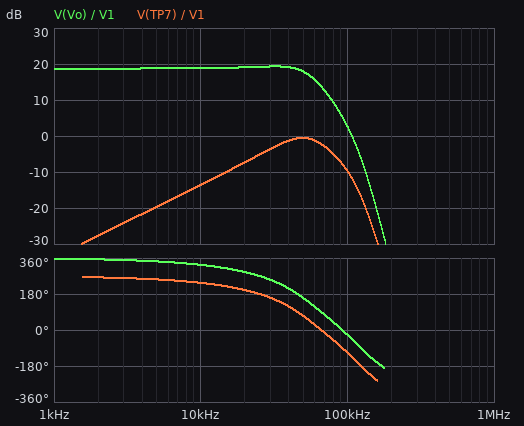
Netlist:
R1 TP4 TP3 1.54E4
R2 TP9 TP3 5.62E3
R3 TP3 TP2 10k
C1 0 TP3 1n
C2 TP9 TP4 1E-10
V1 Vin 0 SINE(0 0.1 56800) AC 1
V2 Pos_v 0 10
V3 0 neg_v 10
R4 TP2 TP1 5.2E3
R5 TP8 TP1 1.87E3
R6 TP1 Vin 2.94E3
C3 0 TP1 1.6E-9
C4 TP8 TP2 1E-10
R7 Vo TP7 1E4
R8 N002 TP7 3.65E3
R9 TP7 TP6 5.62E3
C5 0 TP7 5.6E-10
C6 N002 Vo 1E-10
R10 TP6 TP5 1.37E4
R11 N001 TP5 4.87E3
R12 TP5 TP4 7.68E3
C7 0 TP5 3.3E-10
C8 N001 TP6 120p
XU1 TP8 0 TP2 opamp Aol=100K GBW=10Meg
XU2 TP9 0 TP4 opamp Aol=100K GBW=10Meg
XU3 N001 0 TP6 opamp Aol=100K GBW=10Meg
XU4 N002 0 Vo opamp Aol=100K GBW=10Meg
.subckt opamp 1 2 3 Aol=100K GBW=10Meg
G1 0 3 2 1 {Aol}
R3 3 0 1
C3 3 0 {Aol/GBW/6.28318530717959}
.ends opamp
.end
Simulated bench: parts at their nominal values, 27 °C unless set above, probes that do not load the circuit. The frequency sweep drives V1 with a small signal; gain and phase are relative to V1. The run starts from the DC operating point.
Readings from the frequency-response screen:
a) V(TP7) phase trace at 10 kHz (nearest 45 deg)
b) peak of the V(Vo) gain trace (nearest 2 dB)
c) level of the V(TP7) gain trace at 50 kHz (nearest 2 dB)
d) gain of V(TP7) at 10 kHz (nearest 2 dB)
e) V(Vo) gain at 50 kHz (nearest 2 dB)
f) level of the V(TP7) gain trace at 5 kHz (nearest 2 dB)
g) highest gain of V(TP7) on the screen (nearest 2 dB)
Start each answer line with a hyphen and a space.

- 225 deg
- 20 dB
- 0 dB
- -14 dB
- 18 dB
- -20 dB
- 0 dB
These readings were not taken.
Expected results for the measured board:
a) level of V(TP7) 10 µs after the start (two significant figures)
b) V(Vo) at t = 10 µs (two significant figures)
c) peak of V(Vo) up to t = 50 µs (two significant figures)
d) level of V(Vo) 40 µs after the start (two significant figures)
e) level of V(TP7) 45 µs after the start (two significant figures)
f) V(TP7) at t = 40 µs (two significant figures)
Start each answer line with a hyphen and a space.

- -36 mV
- 210 mV
- 670 mV
- -490 mV
- -78 mV
- 60 mV
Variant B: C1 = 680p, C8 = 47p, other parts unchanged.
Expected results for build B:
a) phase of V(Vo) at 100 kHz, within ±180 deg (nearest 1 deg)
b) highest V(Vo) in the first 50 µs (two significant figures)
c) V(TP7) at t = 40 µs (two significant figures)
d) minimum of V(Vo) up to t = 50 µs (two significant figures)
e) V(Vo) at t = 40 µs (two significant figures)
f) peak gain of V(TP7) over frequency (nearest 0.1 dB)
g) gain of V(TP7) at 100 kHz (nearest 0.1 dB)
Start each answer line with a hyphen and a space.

- 29 deg
- 900 mV
- -20 mV
- -900 mV
- -890 mV
- 2.1 dB
- -0.8 dB
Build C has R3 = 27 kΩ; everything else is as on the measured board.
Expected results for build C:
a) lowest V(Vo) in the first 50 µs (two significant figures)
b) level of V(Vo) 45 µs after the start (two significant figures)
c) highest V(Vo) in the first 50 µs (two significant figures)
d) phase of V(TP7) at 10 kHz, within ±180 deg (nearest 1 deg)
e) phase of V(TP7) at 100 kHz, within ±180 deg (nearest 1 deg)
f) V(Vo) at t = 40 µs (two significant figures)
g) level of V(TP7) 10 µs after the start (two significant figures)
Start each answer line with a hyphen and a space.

- -300 mV
- -160 mV
- 300 mV
- -122 deg
- -119 deg
- -220 mV
- -14 mV
